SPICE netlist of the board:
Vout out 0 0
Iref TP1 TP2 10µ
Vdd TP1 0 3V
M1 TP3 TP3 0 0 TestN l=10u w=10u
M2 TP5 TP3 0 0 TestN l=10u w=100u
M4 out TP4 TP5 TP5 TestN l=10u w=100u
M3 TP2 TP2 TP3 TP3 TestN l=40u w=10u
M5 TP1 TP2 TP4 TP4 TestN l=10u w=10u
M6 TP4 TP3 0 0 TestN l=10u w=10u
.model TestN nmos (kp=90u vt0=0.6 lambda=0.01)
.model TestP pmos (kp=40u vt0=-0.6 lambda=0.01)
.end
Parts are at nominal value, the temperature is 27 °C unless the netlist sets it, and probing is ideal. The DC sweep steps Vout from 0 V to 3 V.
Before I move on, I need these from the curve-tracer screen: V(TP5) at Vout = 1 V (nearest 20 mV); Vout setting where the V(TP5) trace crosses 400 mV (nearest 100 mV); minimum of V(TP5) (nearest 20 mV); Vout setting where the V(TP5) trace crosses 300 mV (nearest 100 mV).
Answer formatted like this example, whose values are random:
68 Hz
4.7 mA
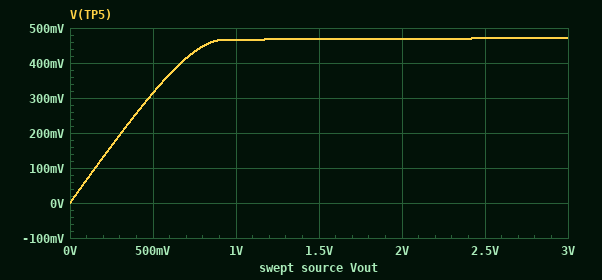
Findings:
460 mV
700 mV
0 V
500 mV
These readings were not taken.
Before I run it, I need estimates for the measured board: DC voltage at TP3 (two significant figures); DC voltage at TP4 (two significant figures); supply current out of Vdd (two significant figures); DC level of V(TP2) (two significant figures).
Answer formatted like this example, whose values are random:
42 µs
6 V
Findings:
1.1 V
1.5 V
20 µA
2.6 V
